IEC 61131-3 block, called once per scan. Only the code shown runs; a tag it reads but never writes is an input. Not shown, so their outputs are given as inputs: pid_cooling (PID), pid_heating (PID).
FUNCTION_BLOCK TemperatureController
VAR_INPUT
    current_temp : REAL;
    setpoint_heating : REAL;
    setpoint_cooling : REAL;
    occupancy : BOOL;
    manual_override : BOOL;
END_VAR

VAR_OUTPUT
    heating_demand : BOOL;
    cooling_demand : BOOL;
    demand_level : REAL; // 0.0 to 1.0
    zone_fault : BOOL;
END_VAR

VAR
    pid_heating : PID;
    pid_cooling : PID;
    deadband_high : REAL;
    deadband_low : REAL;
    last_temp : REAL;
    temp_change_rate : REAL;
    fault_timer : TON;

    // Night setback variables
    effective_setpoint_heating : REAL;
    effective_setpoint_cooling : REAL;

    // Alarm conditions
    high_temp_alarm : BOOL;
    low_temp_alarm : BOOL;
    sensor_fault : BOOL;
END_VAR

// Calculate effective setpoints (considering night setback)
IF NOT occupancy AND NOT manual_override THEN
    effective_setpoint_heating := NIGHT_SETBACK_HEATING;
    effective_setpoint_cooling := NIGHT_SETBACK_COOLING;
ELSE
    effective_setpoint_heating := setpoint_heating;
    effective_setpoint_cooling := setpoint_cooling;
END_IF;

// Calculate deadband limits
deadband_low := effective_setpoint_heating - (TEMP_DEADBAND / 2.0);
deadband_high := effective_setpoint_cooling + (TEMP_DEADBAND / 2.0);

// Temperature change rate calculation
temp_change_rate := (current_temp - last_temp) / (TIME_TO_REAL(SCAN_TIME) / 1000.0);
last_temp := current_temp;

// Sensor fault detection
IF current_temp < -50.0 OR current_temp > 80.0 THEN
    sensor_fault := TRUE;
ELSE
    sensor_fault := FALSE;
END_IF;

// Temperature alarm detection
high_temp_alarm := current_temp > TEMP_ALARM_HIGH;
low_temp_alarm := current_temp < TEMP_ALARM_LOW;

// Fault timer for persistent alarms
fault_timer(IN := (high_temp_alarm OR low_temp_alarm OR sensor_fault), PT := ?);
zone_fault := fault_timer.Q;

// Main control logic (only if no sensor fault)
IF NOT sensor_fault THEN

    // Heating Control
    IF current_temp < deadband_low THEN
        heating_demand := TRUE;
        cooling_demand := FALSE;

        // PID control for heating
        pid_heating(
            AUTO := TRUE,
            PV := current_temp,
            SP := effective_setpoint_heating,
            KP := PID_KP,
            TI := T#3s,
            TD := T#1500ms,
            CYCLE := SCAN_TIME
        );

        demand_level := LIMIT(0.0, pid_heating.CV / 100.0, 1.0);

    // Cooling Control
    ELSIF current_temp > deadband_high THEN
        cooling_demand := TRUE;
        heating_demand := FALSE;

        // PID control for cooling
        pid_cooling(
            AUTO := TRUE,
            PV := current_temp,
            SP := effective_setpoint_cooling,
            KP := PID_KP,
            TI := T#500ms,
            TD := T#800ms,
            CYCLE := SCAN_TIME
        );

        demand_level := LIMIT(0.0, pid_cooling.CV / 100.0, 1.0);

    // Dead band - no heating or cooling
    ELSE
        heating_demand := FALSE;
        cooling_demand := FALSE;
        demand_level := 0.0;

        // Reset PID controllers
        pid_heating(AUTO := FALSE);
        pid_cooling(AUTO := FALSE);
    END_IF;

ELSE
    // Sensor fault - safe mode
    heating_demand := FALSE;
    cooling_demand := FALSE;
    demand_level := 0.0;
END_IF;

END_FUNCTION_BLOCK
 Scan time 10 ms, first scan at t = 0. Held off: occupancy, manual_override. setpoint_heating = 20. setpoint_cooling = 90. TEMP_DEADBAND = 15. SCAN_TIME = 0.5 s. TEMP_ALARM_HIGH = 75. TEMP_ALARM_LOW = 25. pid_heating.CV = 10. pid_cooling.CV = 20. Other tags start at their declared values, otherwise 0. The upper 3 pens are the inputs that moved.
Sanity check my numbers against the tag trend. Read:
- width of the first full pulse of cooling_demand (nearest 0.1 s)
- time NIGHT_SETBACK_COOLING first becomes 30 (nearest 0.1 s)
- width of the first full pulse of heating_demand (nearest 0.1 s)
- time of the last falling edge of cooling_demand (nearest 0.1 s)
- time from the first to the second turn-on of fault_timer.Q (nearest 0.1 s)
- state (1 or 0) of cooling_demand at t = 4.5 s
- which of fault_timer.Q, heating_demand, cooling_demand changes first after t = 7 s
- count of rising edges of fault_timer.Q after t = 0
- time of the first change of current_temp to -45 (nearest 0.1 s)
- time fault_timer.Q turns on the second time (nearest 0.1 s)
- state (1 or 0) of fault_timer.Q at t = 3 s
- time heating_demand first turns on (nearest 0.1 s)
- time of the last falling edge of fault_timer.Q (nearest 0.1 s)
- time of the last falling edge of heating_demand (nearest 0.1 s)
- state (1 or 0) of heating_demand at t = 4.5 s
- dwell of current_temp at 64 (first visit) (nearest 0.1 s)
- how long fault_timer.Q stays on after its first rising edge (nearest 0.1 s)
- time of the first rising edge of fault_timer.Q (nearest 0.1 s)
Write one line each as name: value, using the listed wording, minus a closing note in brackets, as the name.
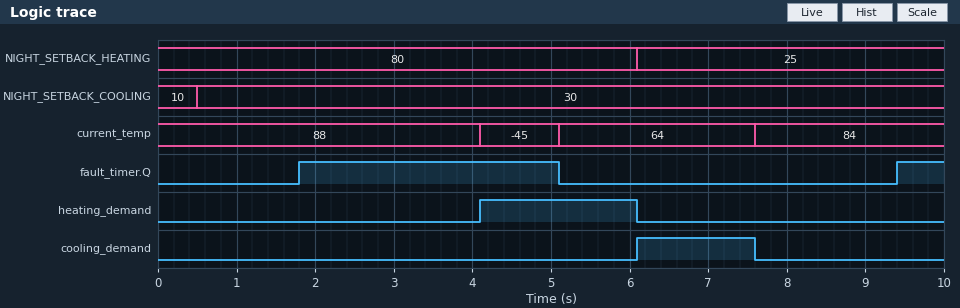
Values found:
width of the first full pulse of cooling_demand: 1.5 s
time NIGHT_SETBACK_COOLING first becomes 30: 0.5 s
width of the first full pulse of heating_demand: 2.0 s
time of the last falling edge of cooling_demand: 7.6 s
time from the first to the second turn-on of fault_timer.Q: 7.6 s
state (1 or 0) of cooling_demand at t = 4.5 s: 0
which of fault_timer.Q, heating_demand, cooling_demand changes first after t = 7 s: cooling_demand
count of rising edges of fault_timer.Q after t = 0: 2
time of the first change of current_temp to -45: 4.1 s
time fault_timer.Q turns on the second time: 9.4 s
state (1 or 0) of fault_timer.Q at t = 3 s: 1
time heating_demand first turns on: 4.1 s
time of the last falling edge of fault_timer.Q: 5.1 s
time of the last falling edge of heating_demand: 6.1 s
state (1 or 0) of heating_demand at t = 4.5 s: 1
dwell of current_temp at 64 (first visit): 2.5 s
how long fault_timer.Q stays on after its first rising edge: 3.3 s
time of the first rising edge of fault_timer.Q: 1.8 s
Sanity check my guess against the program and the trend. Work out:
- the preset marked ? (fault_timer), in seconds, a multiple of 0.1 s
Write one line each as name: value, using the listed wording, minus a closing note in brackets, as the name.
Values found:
the preset marked ? (fault_timer), in seconds, a multiple of 0.1 s: 1.8 s
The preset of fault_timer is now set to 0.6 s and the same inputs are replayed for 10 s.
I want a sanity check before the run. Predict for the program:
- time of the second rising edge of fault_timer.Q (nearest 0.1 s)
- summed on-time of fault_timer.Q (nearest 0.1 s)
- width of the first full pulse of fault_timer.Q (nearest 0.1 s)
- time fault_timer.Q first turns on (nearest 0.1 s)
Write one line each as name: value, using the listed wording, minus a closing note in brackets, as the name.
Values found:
time of the second rising edge of fault_timer.Q: 8.2 s
summed on-time of fault_timer.Q: 6.3 s
width of the first full pulse of fault_timer.Q: 4.5 s
time fault_timer.Q first turns on: 0.6 s
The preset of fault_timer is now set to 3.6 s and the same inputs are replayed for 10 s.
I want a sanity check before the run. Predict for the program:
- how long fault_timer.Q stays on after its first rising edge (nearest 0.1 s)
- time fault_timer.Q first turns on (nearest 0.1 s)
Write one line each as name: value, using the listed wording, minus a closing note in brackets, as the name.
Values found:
how long fault_timer.Q stays on after its first rising edge: 1.5 s
time fault_timer.Q first turns on: 3.6 s
